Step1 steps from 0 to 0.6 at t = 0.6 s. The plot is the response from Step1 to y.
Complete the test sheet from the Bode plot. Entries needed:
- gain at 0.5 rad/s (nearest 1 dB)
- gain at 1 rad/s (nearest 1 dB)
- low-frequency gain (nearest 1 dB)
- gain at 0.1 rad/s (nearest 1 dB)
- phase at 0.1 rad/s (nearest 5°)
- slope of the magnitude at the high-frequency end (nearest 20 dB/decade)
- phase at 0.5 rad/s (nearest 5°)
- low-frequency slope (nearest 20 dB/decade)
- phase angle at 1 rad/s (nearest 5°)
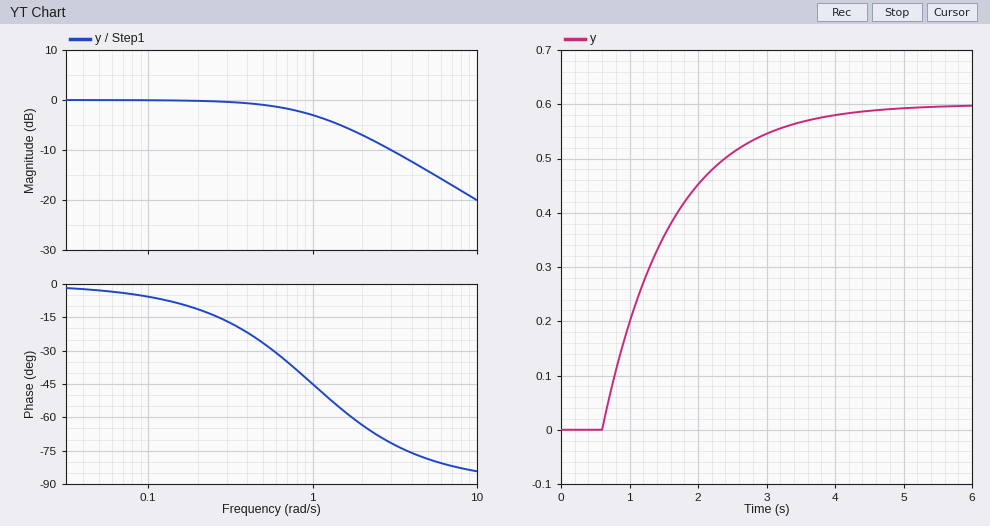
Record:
-1 dB
-3 dB
0 dB
0 dB
-5°
-20 dB/decade
-25°
0 dB/decade
-45°
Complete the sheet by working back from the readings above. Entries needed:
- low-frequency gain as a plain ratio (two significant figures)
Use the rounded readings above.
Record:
1.0
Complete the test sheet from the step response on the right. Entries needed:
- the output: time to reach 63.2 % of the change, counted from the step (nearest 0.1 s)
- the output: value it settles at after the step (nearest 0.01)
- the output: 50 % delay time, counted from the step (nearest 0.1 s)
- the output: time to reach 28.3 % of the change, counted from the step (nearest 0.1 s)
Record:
1.0 s
0.60
0.7 s
0.3 s
